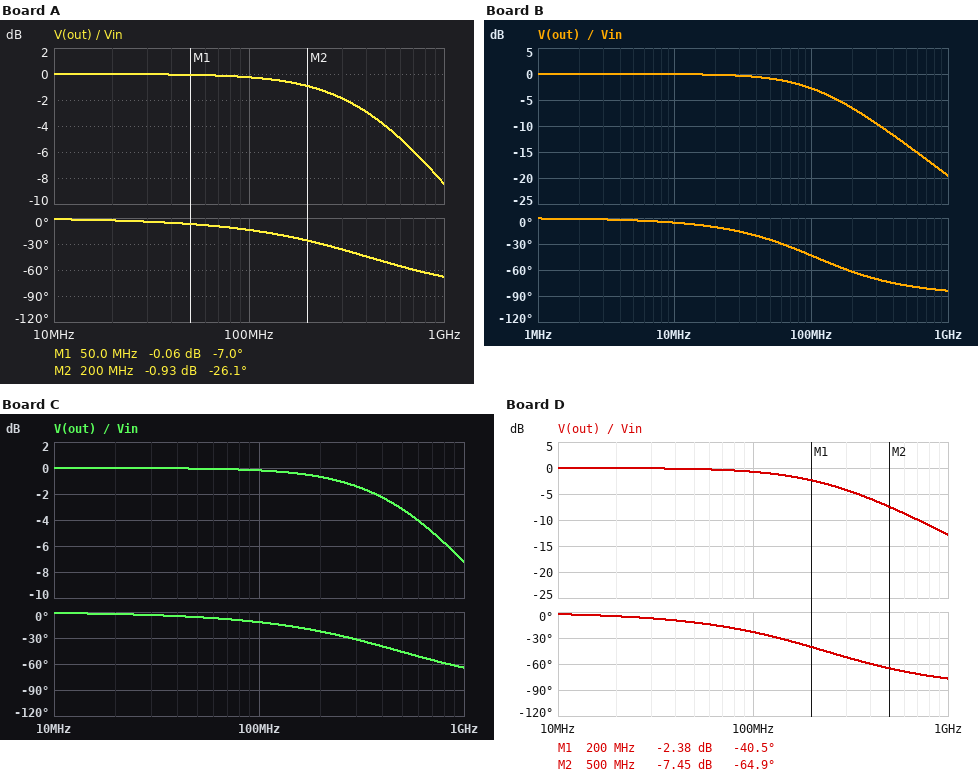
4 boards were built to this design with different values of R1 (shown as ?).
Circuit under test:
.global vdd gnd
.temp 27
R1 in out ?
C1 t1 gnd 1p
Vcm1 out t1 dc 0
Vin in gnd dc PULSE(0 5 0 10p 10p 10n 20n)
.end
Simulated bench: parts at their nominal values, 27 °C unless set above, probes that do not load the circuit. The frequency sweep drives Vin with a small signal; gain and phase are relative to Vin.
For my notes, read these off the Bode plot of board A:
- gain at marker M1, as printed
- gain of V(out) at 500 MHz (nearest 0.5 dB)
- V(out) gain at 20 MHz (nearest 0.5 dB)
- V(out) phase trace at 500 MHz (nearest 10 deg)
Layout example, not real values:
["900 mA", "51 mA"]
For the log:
["-0.06 dB", "-4.0 dB", "0 dB", "-50 deg"]
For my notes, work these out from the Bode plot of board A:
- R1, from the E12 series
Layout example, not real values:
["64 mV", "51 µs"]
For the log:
["390 Ω"]
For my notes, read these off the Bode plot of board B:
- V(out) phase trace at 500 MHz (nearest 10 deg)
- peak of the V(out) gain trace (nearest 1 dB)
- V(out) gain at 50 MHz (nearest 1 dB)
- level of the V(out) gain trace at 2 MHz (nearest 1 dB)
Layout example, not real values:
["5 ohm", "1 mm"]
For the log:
["-80 deg", "0 dB", "-1 dB", "0 dB"]
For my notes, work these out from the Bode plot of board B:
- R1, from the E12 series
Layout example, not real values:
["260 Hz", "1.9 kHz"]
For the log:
["1.5 kΩ"]
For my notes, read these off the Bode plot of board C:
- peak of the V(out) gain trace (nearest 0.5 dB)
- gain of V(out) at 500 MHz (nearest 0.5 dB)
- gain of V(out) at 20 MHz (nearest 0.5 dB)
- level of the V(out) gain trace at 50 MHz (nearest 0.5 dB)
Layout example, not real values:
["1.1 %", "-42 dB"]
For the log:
["0 dB", "-3.0 dB", "0 dB", "0 dB"]
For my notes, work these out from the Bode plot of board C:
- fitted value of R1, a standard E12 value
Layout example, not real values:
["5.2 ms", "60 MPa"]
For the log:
["330 Ω"]
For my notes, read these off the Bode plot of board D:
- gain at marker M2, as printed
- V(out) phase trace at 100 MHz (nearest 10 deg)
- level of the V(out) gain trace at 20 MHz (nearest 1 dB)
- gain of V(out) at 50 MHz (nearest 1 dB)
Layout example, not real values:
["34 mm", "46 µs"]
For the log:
["-7.45 dB", "-20 deg", "0 dB", "0 dB"]
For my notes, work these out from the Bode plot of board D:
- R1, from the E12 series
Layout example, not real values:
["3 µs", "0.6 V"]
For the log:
["680 Ω"]
